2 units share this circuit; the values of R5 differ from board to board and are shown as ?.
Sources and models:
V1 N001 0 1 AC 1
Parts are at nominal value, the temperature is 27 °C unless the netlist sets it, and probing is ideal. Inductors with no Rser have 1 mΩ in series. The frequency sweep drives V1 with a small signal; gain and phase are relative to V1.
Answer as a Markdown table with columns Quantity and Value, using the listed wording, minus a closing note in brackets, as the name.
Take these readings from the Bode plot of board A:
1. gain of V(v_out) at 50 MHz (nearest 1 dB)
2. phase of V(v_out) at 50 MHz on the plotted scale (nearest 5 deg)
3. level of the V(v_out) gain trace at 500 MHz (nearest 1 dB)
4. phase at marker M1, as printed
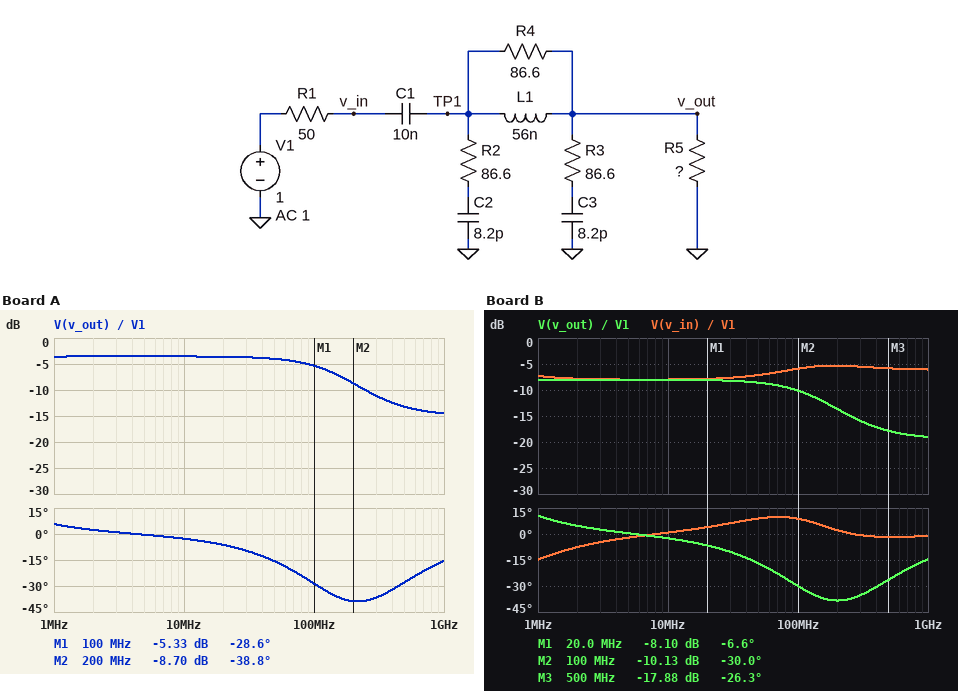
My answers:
| Quantity | Value |
|---|---|
| gain of V(v_out) at 50 MHz | -4 dB |
| phase of V(v_out) at 50 MHz on the plotted scale | -15 deg |
| level of the V(v_out) gain trace at 500 MHz | -13 dB |
| phase at marker M1, as printed | -28.6 deg |
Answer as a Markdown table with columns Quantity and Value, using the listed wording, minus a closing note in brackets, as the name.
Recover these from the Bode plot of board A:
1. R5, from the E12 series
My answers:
| Quantity | Value |
|---|---|
| R5, from the E12 series | 100 Ω |
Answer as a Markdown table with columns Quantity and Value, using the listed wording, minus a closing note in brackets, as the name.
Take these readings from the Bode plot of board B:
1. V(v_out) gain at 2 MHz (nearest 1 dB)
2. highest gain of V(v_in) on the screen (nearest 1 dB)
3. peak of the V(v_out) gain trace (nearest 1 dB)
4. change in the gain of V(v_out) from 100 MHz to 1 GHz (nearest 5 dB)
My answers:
| Quantity | Value |
|---|---|
| V(v_out) gain at 2 MHz | -8 dB |
| highest gain of V(v_in) on the screen | -5 dB |
| peak of the V(v_out) gain trace | -8 dB |
| change in the gain of V(v_out) from 100 MHz to 1 GHz | -10 dB |
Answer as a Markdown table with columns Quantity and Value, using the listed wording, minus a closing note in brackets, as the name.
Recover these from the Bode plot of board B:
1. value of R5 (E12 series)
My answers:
| Quantity | Value |
|---|---|
| value of R5 | 33 Ω |
